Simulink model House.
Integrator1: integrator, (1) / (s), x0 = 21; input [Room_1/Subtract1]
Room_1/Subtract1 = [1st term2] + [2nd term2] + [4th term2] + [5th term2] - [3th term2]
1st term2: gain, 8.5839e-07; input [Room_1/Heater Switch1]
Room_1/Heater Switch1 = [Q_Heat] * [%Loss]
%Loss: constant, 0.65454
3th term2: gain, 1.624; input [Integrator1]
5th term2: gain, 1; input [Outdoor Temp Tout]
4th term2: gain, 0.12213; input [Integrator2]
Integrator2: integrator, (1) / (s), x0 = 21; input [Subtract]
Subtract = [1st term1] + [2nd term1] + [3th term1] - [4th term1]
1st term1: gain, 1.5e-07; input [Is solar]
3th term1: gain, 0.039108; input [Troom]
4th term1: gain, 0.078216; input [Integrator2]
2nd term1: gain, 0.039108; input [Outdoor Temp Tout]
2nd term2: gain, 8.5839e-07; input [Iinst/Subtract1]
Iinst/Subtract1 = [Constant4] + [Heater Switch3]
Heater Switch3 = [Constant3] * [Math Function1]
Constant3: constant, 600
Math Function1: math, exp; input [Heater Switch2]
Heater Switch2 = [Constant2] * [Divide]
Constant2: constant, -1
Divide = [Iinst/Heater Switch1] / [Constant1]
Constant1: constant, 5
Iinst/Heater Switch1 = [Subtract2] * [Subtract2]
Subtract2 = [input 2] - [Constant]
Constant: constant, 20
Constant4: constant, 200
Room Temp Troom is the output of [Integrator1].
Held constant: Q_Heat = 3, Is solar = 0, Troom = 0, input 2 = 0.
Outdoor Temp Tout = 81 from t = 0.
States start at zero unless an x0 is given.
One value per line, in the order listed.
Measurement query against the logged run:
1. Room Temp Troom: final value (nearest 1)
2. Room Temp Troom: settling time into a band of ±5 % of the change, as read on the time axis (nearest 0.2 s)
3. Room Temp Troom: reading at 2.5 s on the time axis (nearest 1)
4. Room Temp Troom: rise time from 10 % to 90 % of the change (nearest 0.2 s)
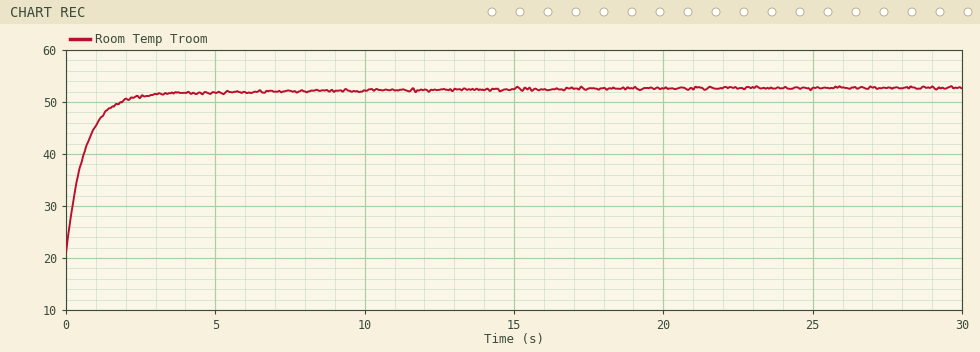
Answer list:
53
2.8 s
51
1.6 s
